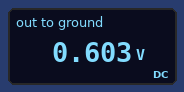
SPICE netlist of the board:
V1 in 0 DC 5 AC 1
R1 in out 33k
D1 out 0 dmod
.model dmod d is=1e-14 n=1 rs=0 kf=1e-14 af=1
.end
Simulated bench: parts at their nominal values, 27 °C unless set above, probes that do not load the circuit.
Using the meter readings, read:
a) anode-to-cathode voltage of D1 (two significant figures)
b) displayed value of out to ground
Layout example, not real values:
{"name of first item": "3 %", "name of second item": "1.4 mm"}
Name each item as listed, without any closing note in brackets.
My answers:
{"anode-to-cathode voltage of D1": "600 mV", "displayed value of out to ground": "0.603 V"}
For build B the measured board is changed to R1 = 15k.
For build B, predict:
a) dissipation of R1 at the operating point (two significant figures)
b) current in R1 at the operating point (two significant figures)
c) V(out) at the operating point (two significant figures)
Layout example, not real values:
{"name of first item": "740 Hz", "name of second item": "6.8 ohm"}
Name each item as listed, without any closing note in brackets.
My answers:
{"dissipation of R1 at the operating point": "1.3 mW", "current in R1 at the operating point": "290 µA", "V(out) at the operating point": "620 mV"}
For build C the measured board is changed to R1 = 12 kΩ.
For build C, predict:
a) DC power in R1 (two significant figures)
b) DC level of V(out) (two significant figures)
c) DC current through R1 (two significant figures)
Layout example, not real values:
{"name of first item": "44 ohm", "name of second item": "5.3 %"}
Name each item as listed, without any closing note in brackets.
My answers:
{"DC power in R1": "1.6 mW", "DC level of V(out)": "630 mV", "DC current through R1": "360 µA"}
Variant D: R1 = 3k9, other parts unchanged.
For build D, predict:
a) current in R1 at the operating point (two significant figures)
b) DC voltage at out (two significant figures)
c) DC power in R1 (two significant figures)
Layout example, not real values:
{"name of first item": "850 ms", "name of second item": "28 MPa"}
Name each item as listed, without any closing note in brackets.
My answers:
{"current in R1 at the operating point": "1.1 mA", "DC voltage at out": "660 mV", "DC power in R1": "4.8 mW"}
